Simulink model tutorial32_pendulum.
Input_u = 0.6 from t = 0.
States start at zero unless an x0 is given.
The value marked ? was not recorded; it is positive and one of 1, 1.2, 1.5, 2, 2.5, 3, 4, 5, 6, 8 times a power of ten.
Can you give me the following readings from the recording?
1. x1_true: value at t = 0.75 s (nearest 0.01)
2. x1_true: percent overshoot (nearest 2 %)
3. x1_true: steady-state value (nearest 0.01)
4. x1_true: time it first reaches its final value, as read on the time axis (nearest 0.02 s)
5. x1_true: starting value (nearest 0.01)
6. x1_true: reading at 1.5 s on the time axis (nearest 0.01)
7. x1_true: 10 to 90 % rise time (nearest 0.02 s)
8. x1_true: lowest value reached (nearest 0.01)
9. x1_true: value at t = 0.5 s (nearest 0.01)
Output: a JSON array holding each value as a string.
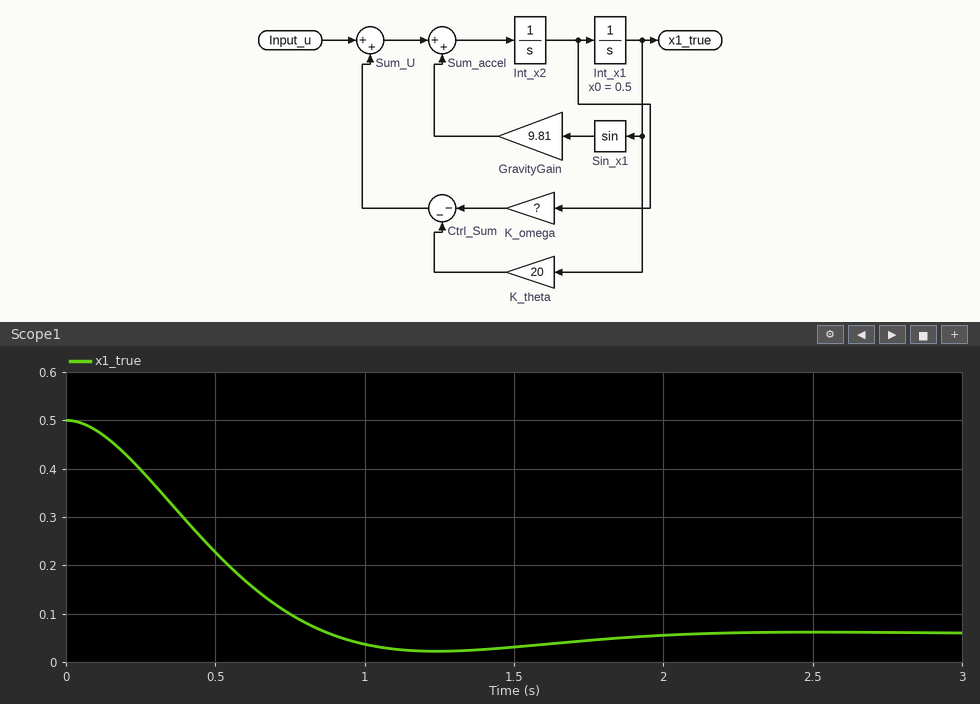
["0.10", "8 %", "0.06", "0.88 s", "0.50", "0.03", "0.58 s", "0.02", "0.23"]
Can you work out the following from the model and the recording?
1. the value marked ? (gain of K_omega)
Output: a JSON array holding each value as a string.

["4"]
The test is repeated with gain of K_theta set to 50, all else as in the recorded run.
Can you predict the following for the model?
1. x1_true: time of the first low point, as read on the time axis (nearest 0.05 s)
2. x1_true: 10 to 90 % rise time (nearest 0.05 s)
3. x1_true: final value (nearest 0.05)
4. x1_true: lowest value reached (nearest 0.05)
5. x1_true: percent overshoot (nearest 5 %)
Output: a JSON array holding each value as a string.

["0.50 s", "0.20 s", "0.00", "-0.15", "35 %"]
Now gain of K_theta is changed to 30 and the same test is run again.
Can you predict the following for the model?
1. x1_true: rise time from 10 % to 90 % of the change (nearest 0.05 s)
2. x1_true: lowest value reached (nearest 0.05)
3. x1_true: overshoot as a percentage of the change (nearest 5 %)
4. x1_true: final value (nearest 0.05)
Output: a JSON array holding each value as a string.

["0.35 s", "-0.05", "20 %", "0.05"]
